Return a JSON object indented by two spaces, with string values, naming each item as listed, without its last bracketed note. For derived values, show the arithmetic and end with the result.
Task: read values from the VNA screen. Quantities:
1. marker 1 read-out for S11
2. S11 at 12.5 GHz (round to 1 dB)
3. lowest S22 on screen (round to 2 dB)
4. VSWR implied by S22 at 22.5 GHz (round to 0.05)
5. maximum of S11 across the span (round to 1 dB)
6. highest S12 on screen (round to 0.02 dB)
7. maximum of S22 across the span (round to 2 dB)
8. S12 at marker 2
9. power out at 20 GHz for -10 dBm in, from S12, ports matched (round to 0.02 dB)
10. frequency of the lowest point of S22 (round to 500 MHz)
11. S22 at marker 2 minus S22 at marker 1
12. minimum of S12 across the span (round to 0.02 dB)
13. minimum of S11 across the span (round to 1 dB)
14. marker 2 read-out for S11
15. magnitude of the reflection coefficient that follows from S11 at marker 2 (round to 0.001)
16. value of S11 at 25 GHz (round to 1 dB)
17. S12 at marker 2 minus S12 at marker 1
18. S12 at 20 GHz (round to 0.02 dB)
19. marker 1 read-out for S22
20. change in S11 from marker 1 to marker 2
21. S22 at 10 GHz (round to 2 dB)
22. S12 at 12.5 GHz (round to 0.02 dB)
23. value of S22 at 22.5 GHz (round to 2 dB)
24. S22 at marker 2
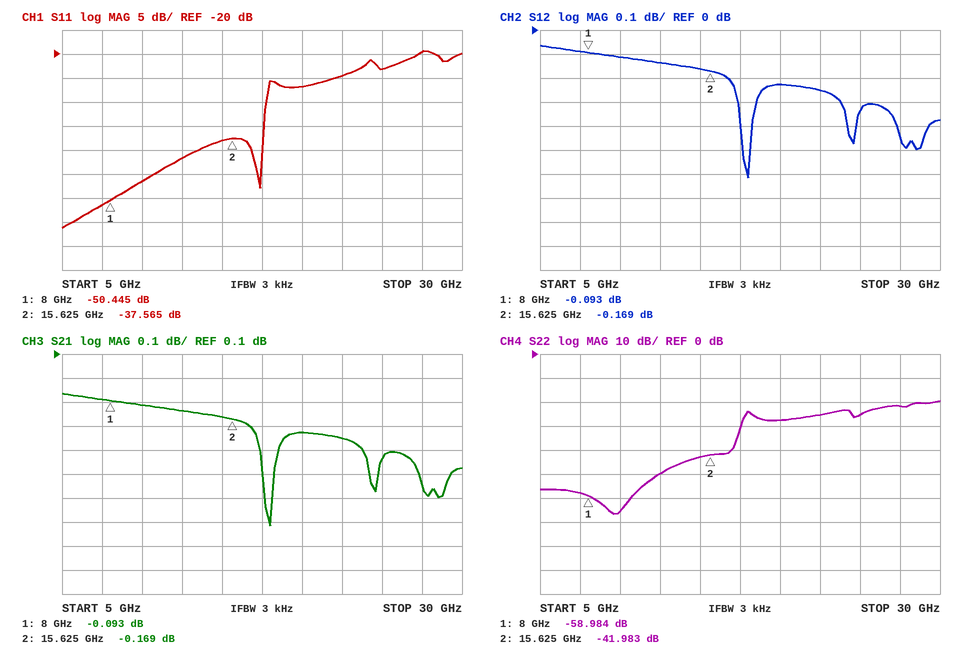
{
  "marker 1 read-out for S11": "-50.445 dB",
  "S11 at 12.5 GHz": "-42 dB",
  "lowest S22 on screen": "-66 dB",
  "VSWR implied by S22 at 22.5 GHz": "|Γ| = 10^(-26/20) = 0.0501; VSWR = (1 + 0.0501)/(1 − 0.0501) ≈ 1.11, so 1.10 to the nearest 0.05",
  "maximum of S11 across the span": "-19 dB",
  "highest S12 on screen": "-0.06 dB",
  "maximum of S22 across the span": "-20 dB",
  "S12 at marker 2": "-0.169 dB",
  "power out at 20 GHz for -10 dBm in, from S12, ports matched": "-10 dBm + (-0.22 dB) = -10.22 dBm",
  "frequency of the lowest point of S22": "9.5 GHz",
  "S22 at marker 2 minus S22 at marker 1": "-41.983 − (-58.984) = 17.001 dB",
  "minimum of S12 across the span": "-0.62 dB",
  "minimum of S11 across the span": "-56 dB",
  "marker 2 read-out for S11": "-37.565 dB",
  "magnitude of the reflection coefficient that follows from S11 at marker 2": "10^(-37.565/20) ≈ 0.013",
  "value of S11 at 25 GHz": "-23 dB",
  "S12 at marker 2 minus S12 at marker 1": "-0.169 − (-0.093) = -0.076 dB",
  "S12 at 20 GHz": "-0.22 dB",
  "marker 1 read-out for S22": "-58.984 dB",
  "change in S11 from marker 1 to marker 2": "-37.565 − (-50.445) = 12.880 dB",
  "S22 at 10 GHz": "-66 dB",
  "S12 at 12.5 GHz": "-0.14 dB",
  "value of S22 at 22.5 GHz": "-26 dB",
  "S22 at marker 2": "-41.983 dB"
}
